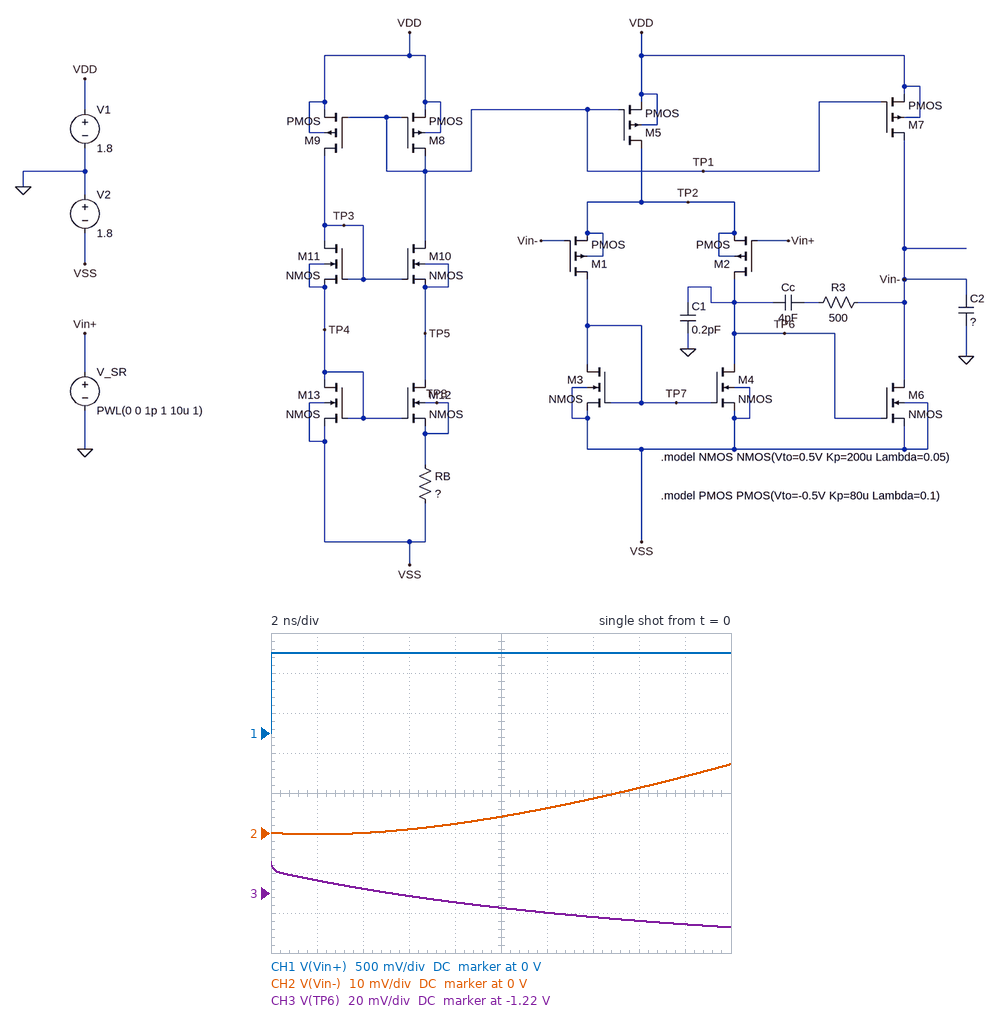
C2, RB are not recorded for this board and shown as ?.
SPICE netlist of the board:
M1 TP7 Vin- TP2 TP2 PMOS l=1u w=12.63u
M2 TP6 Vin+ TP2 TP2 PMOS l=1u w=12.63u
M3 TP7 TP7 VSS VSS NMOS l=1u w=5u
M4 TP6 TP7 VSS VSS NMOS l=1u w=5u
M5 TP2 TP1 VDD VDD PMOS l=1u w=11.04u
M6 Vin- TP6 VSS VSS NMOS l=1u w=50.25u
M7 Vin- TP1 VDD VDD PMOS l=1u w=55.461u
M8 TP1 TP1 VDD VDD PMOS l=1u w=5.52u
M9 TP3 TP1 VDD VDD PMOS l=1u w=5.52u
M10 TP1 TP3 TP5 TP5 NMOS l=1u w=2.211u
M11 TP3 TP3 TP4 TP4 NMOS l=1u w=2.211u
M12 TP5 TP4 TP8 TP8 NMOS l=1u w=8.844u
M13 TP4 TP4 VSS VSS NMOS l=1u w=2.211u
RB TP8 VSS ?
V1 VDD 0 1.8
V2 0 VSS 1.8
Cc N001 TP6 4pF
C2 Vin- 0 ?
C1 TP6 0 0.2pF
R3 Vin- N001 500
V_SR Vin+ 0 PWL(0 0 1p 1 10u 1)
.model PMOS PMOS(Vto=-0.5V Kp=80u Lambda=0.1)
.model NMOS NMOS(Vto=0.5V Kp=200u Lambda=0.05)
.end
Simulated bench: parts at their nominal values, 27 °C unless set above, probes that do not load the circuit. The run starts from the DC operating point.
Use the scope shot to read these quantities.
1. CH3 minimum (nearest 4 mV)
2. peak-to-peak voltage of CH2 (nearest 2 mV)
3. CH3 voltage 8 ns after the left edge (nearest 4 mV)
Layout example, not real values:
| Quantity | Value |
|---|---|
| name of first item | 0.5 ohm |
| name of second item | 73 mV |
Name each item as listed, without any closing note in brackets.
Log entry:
| Quantity | Value |
|---|---|
| CH3 minimum | -1.236 V |
| peak-to-peak voltage of CH2 | 18 mV |
| CH3 voltage 8 ns after the left edge | -1.224 V |
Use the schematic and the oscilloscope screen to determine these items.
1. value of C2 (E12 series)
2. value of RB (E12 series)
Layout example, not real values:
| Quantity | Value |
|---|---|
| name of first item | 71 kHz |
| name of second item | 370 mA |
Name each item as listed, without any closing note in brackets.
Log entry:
| Quantity | Value |
|---|---|
| value of C2 | 12 pF |
| value of RB | 18 kΩ |
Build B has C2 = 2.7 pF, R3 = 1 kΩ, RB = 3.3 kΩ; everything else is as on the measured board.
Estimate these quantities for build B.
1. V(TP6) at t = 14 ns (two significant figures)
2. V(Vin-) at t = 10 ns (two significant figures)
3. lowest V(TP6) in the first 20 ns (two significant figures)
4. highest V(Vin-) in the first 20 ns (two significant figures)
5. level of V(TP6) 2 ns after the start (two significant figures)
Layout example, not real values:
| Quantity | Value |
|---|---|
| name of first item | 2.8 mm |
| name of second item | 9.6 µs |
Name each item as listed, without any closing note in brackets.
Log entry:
| Quantity | Value |
|---|---|
| V(TP6) at t = 14 ns | -920 mV |
| V(Vin-) at t = 10 ns | 490 mV |
| lowest V(TP6) in the first 20 ns | -1.0 V |
| highest V(Vin-) in the first 20 ns | 730 mV |
| level of V(TP6) 2 ns after the start | -940 mV |
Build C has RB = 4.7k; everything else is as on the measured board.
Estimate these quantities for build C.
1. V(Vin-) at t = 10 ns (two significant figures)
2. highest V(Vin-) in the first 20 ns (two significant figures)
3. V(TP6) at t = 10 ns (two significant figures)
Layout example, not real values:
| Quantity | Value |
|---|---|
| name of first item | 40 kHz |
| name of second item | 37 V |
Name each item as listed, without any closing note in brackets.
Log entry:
| Quantity | Value |
|---|---|
| V(Vin-) at t = 10 ns | 170 mV |
| highest V(Vin-) in the first 20 ns | 410 mV |
| V(TP6) at t = 10 ns | -1.1 V |
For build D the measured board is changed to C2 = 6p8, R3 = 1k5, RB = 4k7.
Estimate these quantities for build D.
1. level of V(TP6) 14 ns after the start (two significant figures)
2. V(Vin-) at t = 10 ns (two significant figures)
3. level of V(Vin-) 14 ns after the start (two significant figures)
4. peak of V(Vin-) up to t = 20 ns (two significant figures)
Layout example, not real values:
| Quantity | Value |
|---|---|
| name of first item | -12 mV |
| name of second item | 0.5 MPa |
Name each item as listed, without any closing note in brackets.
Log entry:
| Quantity | Value |
|---|---|
| level of V(TP6) 14 ns after the start | -1.1 V |
| V(Vin-) at t = 10 ns | 310 mV |
| level of V(Vin-) 14 ns after the start | 410 mV |
| peak of V(Vin-) up to t = 20 ns | 560 mV |
